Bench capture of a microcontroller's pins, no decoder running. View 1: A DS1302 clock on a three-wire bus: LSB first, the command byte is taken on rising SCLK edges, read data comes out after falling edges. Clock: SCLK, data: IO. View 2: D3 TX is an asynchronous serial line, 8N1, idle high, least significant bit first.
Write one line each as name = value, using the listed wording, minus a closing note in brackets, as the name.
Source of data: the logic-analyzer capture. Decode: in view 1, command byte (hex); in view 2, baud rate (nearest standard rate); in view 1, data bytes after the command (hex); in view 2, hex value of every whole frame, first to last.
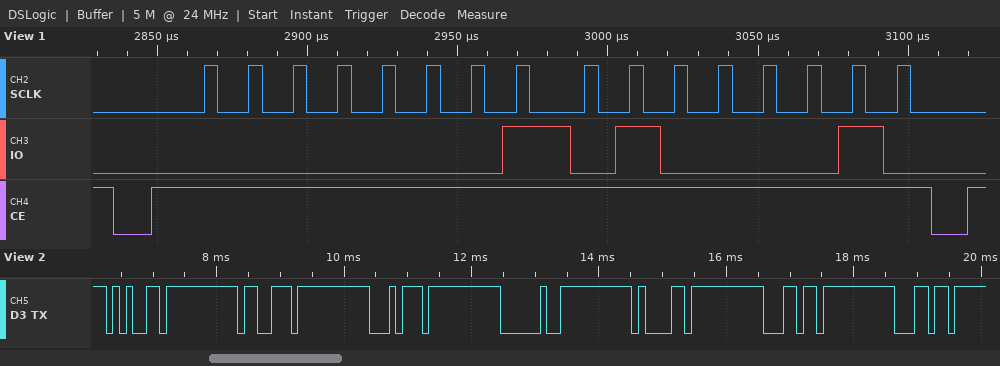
in view 1, command byte = 0x80
in view 2, baud rate = 9600 baud
in view 1, data bytes after the command = 42
in view 2, hex value of every whole frame, first to last = 65 73 74 20 61 6C 6C
